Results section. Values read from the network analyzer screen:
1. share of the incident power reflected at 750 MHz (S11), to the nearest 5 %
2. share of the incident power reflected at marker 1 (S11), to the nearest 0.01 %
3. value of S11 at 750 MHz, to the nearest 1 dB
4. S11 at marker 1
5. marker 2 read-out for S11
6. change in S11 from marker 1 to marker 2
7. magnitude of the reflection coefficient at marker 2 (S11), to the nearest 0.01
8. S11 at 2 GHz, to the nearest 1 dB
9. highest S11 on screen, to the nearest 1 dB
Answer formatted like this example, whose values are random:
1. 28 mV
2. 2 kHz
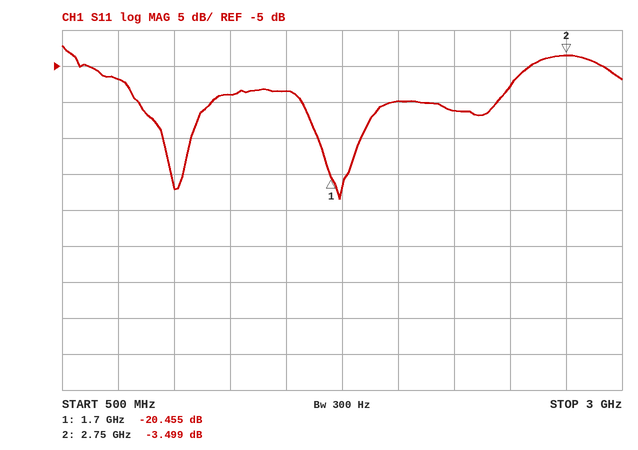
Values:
1. 20 %
2. 0.90 %
3. -7 dB
4. -20.455 dB
5. -3.499 dB
6. 16.956 dB
7. 0.67
8. -10 dB
9. -2 dB
